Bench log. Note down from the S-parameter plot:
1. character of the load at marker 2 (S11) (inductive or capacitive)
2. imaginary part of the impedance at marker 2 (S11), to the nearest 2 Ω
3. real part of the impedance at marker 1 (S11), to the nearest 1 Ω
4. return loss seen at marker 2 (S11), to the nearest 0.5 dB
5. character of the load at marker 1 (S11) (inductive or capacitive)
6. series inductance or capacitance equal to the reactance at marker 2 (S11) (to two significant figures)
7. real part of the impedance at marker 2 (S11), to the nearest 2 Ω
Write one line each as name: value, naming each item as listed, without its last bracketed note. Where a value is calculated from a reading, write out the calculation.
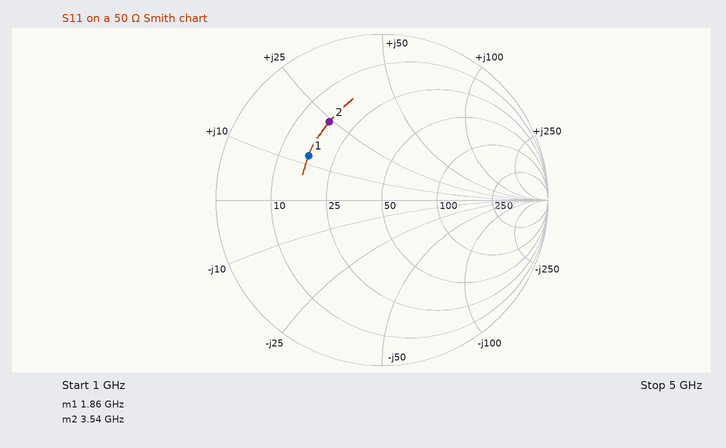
character of the load at marker 2 (S11): inductive
imaginary part of the impedance at marker 2 (S11), to the nearest 2 Ω: +24 Ω
real part of the impedance at marker 1 (S11), to the nearest 1 Ω: 17 Ω
return loss seen at marker 2 (S11), to the nearest 0.5 dB: 5.0 dB
character of the load at marker 1 (S11): inductive
series inductance or capacitance equal to the reactance at marker 2 (S11): L = 24 Ω/(2π × 3.54 GHz) ≈ 1.1 nH
real part of the impedance at marker 2 (S11), to the nearest 2 Ω: 18 Ω
